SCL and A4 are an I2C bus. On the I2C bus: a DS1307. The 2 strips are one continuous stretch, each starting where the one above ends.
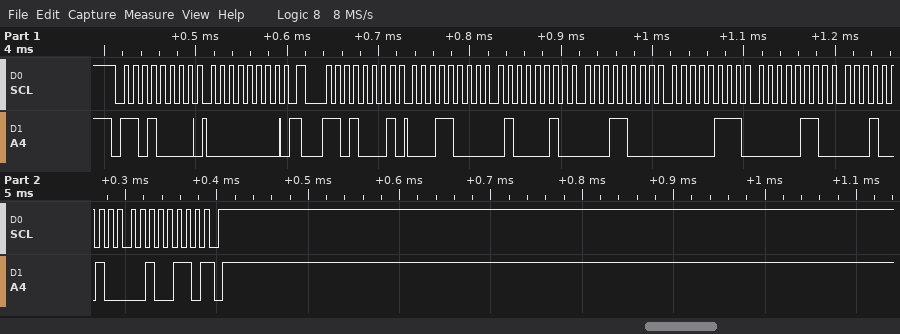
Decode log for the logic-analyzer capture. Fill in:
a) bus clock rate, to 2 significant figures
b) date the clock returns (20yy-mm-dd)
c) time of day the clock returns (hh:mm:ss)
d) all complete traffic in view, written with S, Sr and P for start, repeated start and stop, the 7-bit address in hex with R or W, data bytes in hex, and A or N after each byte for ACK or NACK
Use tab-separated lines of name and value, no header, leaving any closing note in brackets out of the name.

bus clock rate, to 2 significant figures	100 kHz
date the clock returns	2026-12-06
time of day the clock returns	18:42:18
all complete traffic in view, written with S, Sr and P for start, repeated start and stop, the 7-bit address in hex with R or W, data bytes in hex, and A or N after each byte for ACK or NACK	S 68W A 00 A Sr 68R A 18 A 42 A 18 A 07 A 06 A 12 A 26 N P
